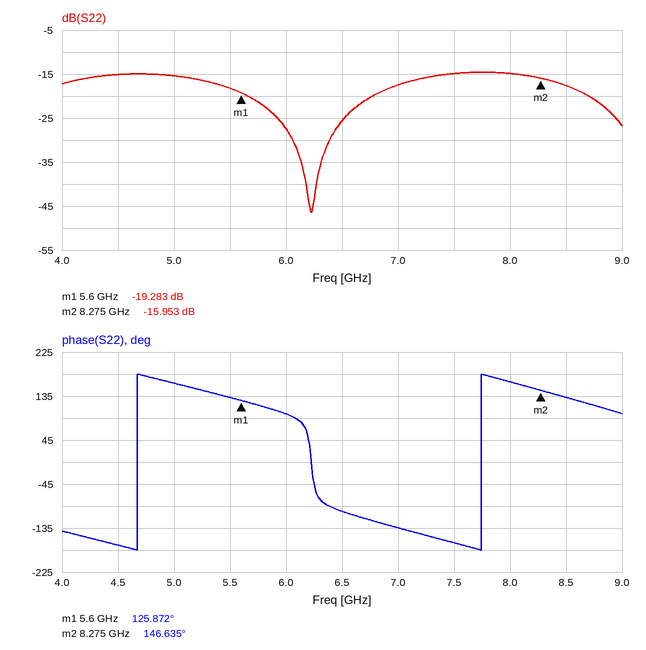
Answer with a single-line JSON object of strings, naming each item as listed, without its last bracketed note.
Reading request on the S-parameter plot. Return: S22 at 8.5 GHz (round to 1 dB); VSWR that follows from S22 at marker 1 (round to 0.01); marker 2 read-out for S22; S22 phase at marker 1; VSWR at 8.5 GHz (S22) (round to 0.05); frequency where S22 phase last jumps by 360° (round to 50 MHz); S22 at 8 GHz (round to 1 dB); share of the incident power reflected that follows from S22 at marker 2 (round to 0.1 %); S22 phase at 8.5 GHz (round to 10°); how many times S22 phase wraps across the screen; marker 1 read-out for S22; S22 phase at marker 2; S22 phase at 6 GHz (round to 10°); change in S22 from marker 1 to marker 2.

{"S22 at 8.5 GHz": "-18 dB", "VSWR that follows from S22 at marker 1": "1.24", "marker 2 read-out for S22": "-15.953 dB", "S22 phase at marker 1": "125.872°", "VSWR at 8.5 GHz (S22)": "1.30", "frequency where S22 phase last jumps by 360°": "7.75 GHz", "S22 at 8 GHz": "-15 dB", "share of the incident power reflected that follows from S22 at marker 2": "2.5 %", "S22 phase at 8.5 GHz": "130°", "how many times S22 phase wraps across the screen": "2", "marker 1 read-out for S22": "-19.283 dB", "S22 phase at marker 2": "146.635°", "S22 phase at 6 GHz": "100°", "change in S22 from marker 1 to marker 2": "3.330 dB"}
